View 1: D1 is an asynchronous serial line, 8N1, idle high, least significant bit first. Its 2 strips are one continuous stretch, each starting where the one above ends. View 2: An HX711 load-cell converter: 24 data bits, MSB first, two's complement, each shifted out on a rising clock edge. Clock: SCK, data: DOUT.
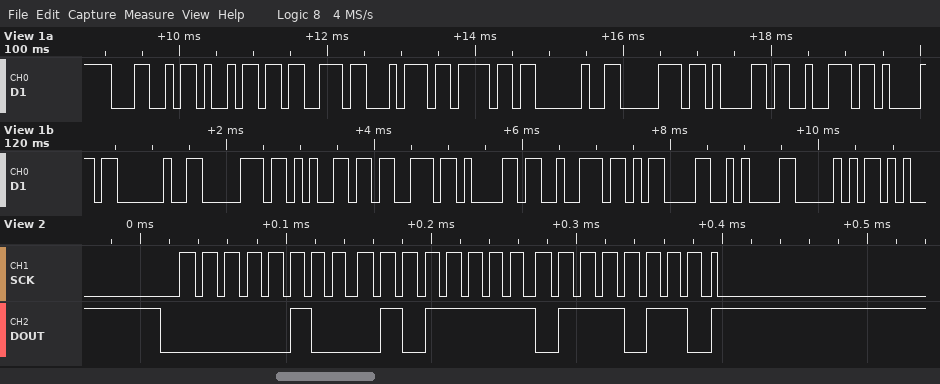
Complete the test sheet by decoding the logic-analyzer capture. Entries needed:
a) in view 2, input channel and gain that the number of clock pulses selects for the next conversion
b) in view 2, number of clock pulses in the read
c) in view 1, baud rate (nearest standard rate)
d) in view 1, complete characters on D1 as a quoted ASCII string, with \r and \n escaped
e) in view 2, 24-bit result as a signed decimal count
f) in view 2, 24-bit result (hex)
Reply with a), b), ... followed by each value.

a) channel A, gain 128
b) 25
c) 9600 baud
d) "Listo para pesar\r\nP"
e) 286582
f) 0x045F76
